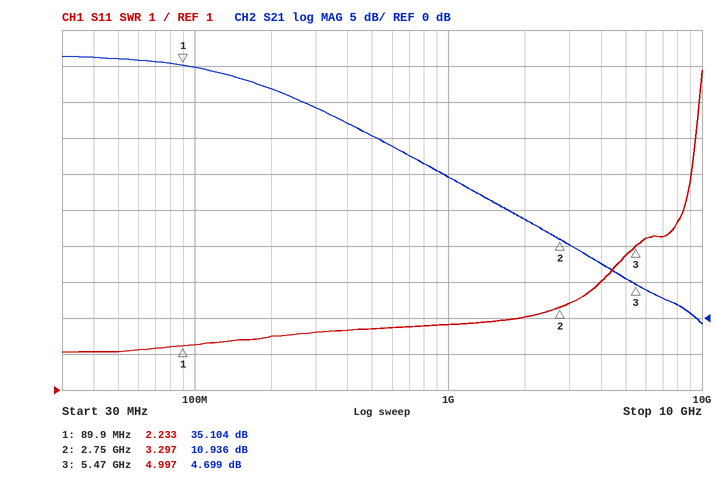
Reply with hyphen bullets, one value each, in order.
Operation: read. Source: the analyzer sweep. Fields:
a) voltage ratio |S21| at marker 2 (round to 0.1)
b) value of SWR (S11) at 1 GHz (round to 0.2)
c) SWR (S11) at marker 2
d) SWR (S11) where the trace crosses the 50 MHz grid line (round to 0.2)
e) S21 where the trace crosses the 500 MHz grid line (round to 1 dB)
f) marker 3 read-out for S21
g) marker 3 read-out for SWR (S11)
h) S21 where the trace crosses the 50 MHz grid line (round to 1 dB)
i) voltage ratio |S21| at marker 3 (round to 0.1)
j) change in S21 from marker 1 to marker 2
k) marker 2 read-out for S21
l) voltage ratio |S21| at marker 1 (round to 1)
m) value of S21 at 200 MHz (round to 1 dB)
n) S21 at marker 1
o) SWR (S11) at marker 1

- 3.5
- 2.8
- 3.297
- 2.0
- 25 dB
- 4.699 dB
- 4.997
- 36 dB
- 1.7
- -24.168 dB
- 10.936 dB
- 57
- 32 dB
- 35.104 dB
- 2.233
